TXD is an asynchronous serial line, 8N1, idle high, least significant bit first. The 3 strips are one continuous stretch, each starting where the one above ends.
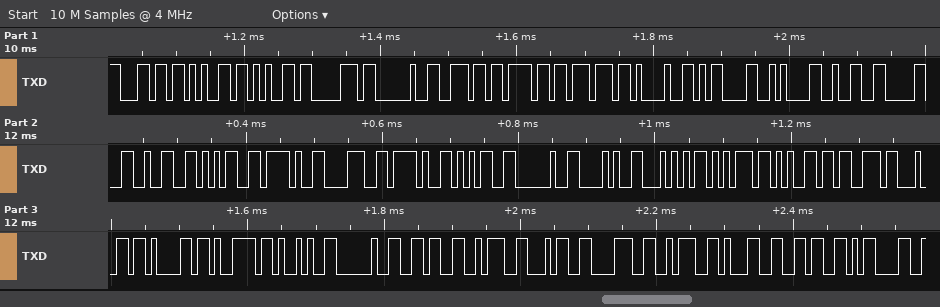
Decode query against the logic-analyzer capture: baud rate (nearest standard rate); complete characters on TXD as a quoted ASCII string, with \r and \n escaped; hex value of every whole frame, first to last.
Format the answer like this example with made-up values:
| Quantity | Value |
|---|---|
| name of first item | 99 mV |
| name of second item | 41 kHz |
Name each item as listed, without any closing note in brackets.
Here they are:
| Quantity | Value |
|---|---|
| baud rate | 115200 baud |
| complete characters on TXD as a quoted ASCII string, with \r and \n escaped | "leep now!\r\n2025/8/5 (Tuesday) 6:48:16\r" |
| hex value of every whole frame, first to last | 0x6C 0x65 0x65 0x70 0x20 0x6E 0x6F 0x77 0x21 0x0D 0x0A 0x32 0x30 0x32 0x35 0x2F 0x38 0x2F 0x35 0x20 0x28 0x54 0x75 0x65 0x73 0x64 0x61 0x79 0x29 0x20 0x36 0x3A 0x34 0x38 0x3A 0x31 0x36 0x0D |
